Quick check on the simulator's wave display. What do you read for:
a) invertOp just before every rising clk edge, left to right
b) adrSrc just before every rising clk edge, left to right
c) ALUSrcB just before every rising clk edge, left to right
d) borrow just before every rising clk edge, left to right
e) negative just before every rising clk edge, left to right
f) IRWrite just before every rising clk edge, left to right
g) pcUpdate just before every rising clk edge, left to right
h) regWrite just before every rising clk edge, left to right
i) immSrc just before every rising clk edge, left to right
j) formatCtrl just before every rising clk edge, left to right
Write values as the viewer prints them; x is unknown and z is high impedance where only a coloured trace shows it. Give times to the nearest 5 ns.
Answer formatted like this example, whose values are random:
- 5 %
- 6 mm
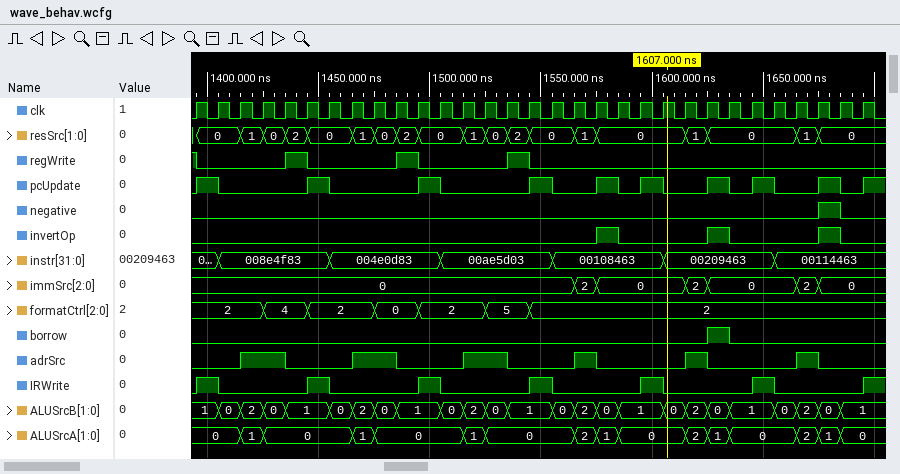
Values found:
- 0 0 0 0 0 0 0 0 0 0 0 0 0 0 0 0 0 0 0 1 0 0 0 0 1 0 0 0 0 1 0
- 0 0 0 1 1 0 0 0 1 1 0 0 0 1 1 0 0 0 1 0 0 0 0 1 0 0 0 0 1 0 0
- 1, 1, 0, 2, 0, 1, 1, 0, 2, 0, 1, 1, 0, 2, 0, 1, 1, 0, 2, 0, 1, 1, 0, 2, 0, 1, 1, 0, 2, 0, 1
- 0 0 0 0 0 0 0 0 0 0 0 0 0 0 0 0 0 0 0 0 0 0 0 0 1 0 0 0 0 0 0
- 0 0 0 0 0 0 0 0 0 0 0 0 0 0 0 0 0 0 0 0 0 0 0 0 0 0 0 0 0 1 0
- 0 1 0 0 0 0 1 0 0 0 0 1 0 0 0 0 1 0 0 0 0 1 0 0 0 0 1 0 0 0 0
- 0 1 0 0 0 0 1 0 0 0 0 1 0 0 0 0 1 0 0 1 0 1 0 0 1 0 1 0 0 1 0
- 1 0 0 0 0 1 0 0 0 0 1 0 0 0 0 1 0 0 0 0 0 0 0 0 0 0 0 0 0 0 0
- 0, 0, 0, 0, 0, 0, 0, 0, 0, 0, 0, 0, 0, 0, 0, 0, 0, 0, 2, 0, 0, 0, 0, 2, 0, 0, 0, 0, 2, 0, 0
- 2, 2, 2, 2, 4, 4, 2, 2, 2, 0, 0, 2, 2, 2, 5, 5, 2, 2, 2, 2, 2, 2, 2, 2, 2, 2, 2, 2, 2, 2, 2
